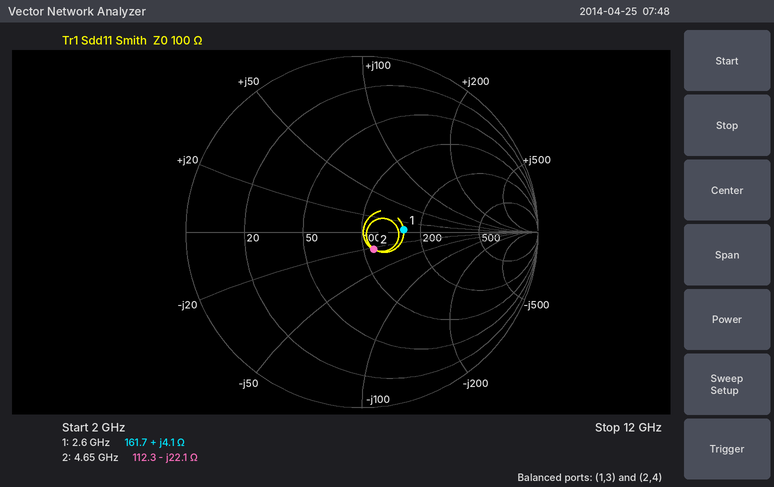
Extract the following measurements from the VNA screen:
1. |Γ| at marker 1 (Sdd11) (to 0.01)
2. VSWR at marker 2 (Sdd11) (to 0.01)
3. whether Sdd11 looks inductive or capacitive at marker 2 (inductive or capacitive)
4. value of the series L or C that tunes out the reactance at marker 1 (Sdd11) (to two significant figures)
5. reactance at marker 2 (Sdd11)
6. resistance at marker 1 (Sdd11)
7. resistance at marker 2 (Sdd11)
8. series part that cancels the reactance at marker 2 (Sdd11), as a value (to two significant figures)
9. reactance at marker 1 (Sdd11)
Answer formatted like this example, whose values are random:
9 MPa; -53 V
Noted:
0.24; 1.27; capacitive; 15 pF; -22.1 Ω; 161.7 Ω; 112.3 Ω; 760 pH; +4.1 Ω
